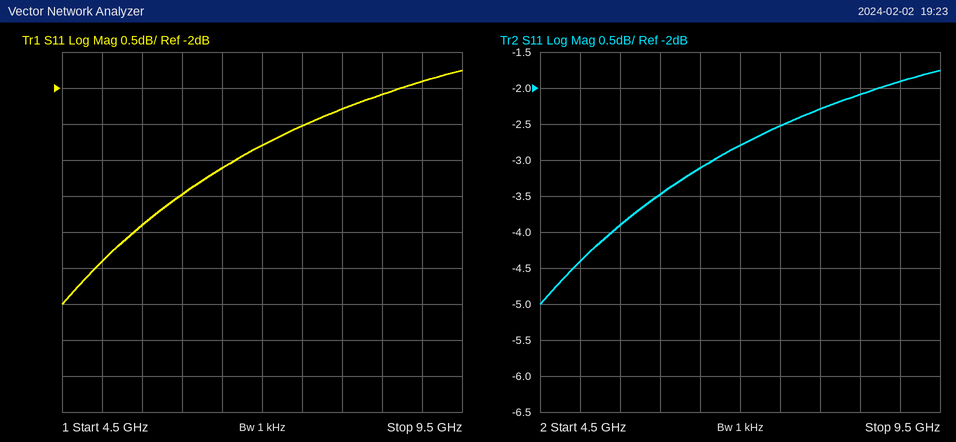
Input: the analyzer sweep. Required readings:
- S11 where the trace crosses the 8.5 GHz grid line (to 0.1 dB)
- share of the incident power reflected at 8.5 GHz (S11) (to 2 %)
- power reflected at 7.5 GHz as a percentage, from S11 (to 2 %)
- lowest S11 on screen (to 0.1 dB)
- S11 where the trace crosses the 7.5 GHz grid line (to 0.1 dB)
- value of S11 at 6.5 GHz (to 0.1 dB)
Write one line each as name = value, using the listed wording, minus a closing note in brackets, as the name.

S11 where the trace crosses the 8.5 GHz grid line = -2.1 dB
share of the incident power reflected at 8.5 GHz (S11) = 62 %
power reflected at 7.5 GHz as a percentage, from S11 = 56 %
lowest S11 on screen = -5.0 dB
S11 where the trace crosses the 7.5 GHz grid line = -2.5 dB
value of S11 at 6.5 GHz = -3.1 dB
